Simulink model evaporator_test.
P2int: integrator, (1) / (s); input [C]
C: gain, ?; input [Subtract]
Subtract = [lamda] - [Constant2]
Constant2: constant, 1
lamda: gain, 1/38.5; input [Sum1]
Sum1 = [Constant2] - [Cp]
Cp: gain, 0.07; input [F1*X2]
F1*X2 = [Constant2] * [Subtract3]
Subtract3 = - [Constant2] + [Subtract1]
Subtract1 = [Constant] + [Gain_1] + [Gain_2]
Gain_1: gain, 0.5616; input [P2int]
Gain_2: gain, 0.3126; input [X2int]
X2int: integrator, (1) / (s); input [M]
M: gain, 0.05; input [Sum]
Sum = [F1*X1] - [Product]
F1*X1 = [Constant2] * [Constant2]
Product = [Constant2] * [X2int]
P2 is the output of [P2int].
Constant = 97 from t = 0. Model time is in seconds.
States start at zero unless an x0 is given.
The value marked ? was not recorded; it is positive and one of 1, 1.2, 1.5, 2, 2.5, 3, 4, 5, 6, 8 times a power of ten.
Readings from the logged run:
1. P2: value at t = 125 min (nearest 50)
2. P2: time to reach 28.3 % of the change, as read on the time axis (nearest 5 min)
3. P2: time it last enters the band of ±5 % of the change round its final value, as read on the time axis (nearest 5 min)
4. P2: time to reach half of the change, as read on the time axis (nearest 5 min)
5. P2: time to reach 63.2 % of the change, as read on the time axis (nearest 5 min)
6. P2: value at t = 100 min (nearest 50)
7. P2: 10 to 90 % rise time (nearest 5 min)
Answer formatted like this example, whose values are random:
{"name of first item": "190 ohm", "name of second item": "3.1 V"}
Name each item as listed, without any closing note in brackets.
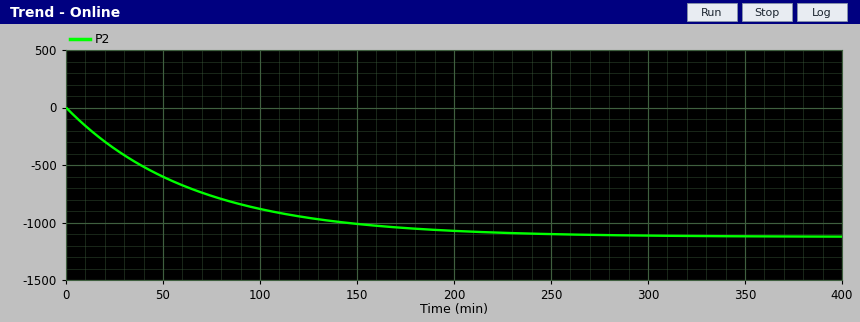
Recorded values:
{"P2: value at t = 125 min": "-950", "P2: time to reach 28.3 % of the change, as read on the time axis": "20 min", "P2: time it last enters the band of ±5 % of the change round its final value, as read on the time axis": "195 min", "P2: time to reach half of the change, as read on the time axis": "45 min", "P2: time to reach 63.2 % of the change, as read on the time axis": "65 min", "P2: value at t = 100 min": "-900", "P2: 10 to 90 % rise time": "145 min"}
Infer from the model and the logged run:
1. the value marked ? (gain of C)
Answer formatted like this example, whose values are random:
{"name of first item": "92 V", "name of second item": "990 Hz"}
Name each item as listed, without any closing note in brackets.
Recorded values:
{"the value marked ?": "0.25"}
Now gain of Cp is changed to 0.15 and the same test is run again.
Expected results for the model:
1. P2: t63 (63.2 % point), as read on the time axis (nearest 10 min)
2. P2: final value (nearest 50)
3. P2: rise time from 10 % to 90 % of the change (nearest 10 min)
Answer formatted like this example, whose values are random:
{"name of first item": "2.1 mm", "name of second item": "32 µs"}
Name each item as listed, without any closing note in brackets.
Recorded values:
{"P2: t63 (63.2 % point), as read on the time axis": "30 min", "P2: final value": "-600", "P2: rise time from 10 % to 90 % of the change": "70 min"}
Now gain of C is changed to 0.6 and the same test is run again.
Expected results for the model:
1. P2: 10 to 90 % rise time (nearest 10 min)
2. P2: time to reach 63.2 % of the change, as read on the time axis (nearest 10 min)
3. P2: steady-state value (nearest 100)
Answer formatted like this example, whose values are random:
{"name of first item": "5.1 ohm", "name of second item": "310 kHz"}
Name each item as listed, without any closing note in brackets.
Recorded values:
{"P2: 10 to 90 % rise time": "60 min", "P2: time to reach 63.2 % of the change, as read on the time axis": "30 min", "P2: steady-state value": "-1100"}
